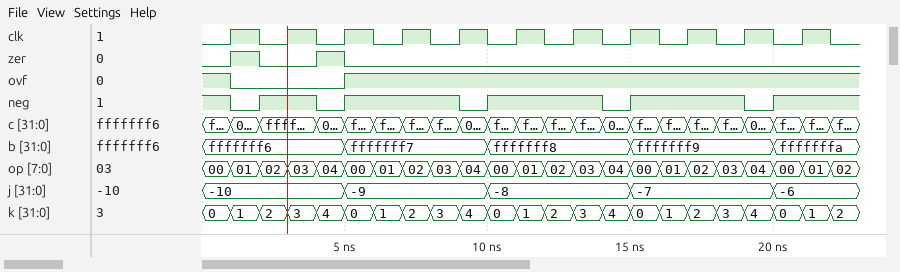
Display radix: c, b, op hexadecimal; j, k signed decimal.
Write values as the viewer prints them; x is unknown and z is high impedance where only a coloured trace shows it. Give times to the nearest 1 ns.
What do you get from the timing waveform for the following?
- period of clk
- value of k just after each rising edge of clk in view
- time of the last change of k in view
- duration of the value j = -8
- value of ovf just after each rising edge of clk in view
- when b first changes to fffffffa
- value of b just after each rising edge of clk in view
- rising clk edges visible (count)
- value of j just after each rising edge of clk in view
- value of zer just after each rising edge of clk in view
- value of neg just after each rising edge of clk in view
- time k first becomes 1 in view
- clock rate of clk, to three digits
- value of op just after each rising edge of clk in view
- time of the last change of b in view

2 ns
1, 3, 0, 2, 4, 1, 3, 0, 2, 4, 1
22 ns
5 ns
0 0 1 1 1 1 1 1 1 1 1
20 ns
fffffff6, fffffff6, fffffff7, fffffff7, fffffff7, fffffff8, fffffff8, fffffff9, fffffff9, fffffff9, fffffffa
11
-10, -10, -9, -9, -9, -8, -8, -7, -7, -7, -6
1 0 0 0 0 0 0 0 0 0 0
0 1 1 1 0 1 1 1 1 0 1
1 ns
500 MHz
01, 03, 00, 02, 04, 01, 03, 00, 02, 04, 01
20 ns
